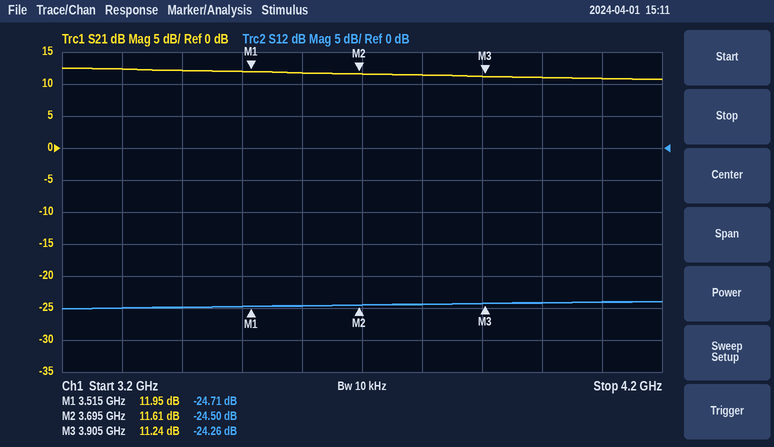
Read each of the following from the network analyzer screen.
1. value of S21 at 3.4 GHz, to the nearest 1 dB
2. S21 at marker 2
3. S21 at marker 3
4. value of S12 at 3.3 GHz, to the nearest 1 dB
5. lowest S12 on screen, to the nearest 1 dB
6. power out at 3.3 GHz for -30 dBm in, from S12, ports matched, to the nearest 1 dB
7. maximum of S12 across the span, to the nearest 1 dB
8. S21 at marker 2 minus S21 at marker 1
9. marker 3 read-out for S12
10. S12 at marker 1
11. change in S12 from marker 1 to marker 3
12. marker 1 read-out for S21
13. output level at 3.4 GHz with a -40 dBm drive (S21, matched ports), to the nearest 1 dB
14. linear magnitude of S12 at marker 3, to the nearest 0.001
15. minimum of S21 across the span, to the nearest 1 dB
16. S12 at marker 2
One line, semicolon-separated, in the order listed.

12 dB; 11.61 dB; 11.24 dB; -25 dB; -25 dB; -55 dBm; -24 dB; -0.34 dB; -24.26 dB; -24.71 dB; 0.45 dB; 11.95 dB; -28 dBm; 0.061; 11 dB; -24.50 dB
